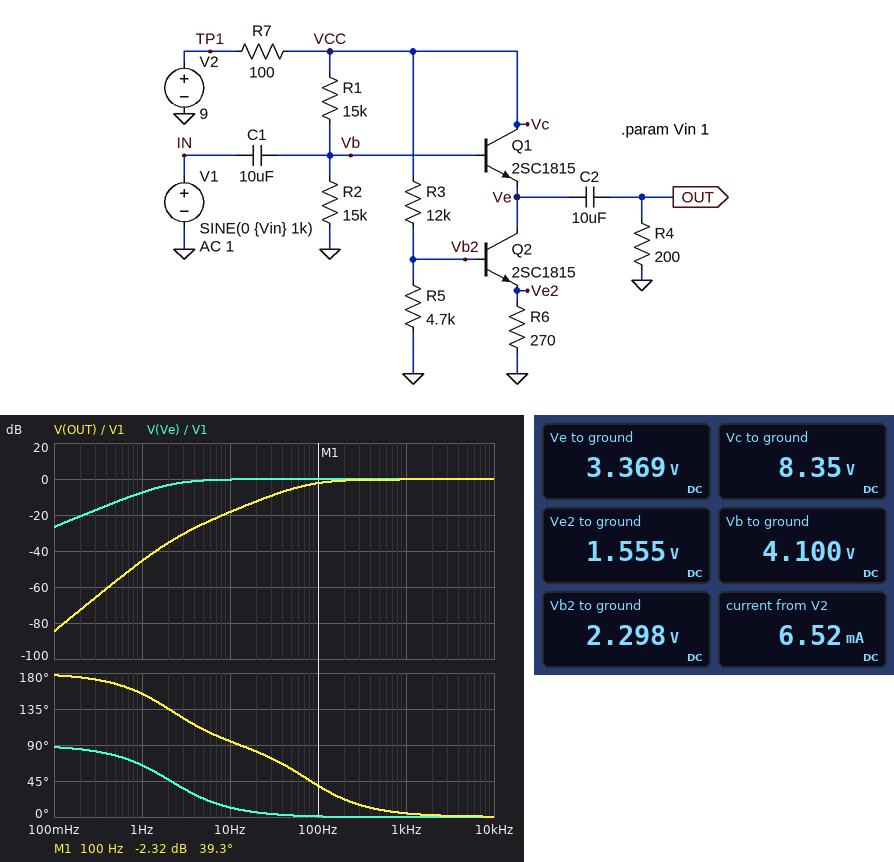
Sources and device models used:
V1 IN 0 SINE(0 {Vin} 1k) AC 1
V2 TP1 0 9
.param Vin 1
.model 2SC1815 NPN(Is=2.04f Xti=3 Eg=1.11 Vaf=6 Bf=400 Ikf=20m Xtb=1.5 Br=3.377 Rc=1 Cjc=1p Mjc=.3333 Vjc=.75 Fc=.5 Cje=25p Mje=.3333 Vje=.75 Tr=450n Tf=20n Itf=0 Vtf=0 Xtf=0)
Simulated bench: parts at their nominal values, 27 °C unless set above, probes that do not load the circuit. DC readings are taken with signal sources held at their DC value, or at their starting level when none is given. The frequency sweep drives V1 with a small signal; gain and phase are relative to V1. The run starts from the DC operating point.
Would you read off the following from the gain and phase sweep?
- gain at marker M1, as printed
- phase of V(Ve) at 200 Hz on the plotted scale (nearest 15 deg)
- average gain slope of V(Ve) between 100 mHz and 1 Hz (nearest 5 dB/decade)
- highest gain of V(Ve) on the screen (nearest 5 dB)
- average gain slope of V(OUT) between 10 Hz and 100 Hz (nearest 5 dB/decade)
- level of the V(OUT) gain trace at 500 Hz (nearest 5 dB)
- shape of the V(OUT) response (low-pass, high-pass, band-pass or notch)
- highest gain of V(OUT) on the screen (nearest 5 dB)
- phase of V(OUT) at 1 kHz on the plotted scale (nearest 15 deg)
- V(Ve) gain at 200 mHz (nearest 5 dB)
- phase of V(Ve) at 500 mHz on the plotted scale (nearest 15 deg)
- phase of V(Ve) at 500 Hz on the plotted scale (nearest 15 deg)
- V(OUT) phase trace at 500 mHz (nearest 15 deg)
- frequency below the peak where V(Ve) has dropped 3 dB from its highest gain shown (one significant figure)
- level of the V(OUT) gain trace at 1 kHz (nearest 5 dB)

-2.32 dB
0 deg
20 dB/decade
0 dB
15 dB/decade
0 dB
high-pass
0 dB
0 deg
-20 dB
75 deg
0 deg
165 deg
2 Hz
0 dB
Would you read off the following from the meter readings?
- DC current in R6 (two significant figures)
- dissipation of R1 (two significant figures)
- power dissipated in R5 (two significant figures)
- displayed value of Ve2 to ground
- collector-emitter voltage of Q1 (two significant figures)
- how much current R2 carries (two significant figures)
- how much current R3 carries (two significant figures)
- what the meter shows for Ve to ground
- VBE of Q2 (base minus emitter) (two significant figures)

5.8 mA
1.2 mW
1.1 mW
1.555 V
5.0 V
270 µA
500 µA
3.369 V
740 mV
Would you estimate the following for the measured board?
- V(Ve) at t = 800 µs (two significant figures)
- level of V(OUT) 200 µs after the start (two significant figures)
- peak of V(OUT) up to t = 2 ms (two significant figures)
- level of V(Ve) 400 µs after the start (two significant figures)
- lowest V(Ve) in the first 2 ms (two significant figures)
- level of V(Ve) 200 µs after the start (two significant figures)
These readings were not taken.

2.5 V
880 mV
930 mV
3.9 V
2.4 V
4.3 V
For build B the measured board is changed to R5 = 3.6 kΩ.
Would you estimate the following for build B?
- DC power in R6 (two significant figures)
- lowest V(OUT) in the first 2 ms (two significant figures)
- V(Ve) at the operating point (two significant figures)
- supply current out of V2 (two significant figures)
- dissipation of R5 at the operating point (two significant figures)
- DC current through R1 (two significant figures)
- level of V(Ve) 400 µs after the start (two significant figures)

5.3 mW
-930 mV
3.5 V
5.2 mA
1.0 mW
290 µA
4.0 V
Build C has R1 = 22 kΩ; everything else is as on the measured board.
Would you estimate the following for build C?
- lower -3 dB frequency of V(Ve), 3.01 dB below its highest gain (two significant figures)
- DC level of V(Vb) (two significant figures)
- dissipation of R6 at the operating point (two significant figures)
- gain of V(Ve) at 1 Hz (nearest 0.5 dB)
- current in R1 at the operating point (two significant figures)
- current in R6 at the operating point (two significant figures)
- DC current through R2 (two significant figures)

1.8 Hz
3.3 V
8.9 mW
-6.5 dB
230 µA
5.7 mA
220 µA
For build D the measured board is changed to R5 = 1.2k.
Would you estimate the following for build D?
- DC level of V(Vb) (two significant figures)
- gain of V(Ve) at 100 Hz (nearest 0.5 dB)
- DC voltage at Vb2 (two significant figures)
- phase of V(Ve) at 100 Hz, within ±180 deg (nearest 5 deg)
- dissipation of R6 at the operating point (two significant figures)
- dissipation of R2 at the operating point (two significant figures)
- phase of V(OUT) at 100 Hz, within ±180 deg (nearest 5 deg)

4.4 V
-1.5 dB
800 mV
-5 deg
68 µW
1.3 mW
35 deg
